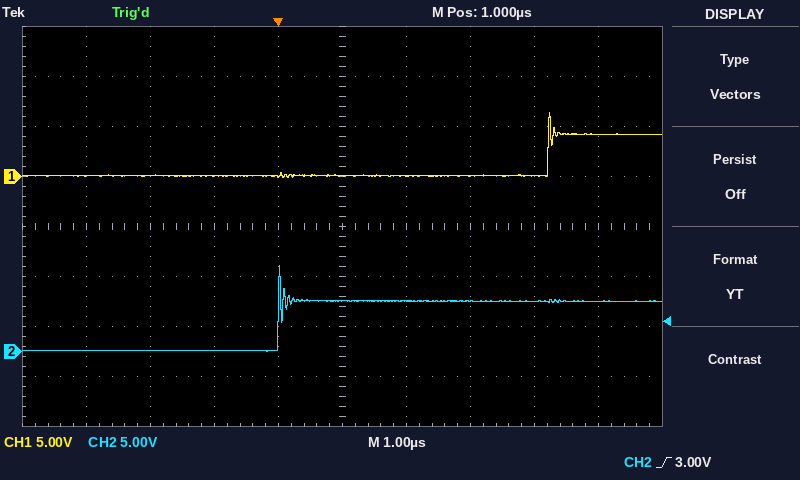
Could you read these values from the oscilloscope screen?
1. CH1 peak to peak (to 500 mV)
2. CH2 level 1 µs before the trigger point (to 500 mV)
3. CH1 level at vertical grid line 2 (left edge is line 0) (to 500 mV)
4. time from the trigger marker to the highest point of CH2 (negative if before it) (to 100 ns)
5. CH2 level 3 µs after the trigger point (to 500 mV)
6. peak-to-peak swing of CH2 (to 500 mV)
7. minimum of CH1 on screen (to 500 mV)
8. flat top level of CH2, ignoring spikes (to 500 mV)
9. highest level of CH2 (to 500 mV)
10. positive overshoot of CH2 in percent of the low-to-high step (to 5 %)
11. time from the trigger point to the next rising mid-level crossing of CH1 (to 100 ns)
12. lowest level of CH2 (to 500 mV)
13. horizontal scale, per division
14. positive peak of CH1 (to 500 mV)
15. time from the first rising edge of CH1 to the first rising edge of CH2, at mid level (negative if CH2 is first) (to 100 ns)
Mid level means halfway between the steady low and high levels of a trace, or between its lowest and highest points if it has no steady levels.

6.5 V
0.0 V
0.0 V
0.0 µs
5.0 V
8.5 V
0.0 V
5.0 V
8.5 V
70 %
4.2 µs
0.0 V
1 µs
6.5 V
-4.2 µs
